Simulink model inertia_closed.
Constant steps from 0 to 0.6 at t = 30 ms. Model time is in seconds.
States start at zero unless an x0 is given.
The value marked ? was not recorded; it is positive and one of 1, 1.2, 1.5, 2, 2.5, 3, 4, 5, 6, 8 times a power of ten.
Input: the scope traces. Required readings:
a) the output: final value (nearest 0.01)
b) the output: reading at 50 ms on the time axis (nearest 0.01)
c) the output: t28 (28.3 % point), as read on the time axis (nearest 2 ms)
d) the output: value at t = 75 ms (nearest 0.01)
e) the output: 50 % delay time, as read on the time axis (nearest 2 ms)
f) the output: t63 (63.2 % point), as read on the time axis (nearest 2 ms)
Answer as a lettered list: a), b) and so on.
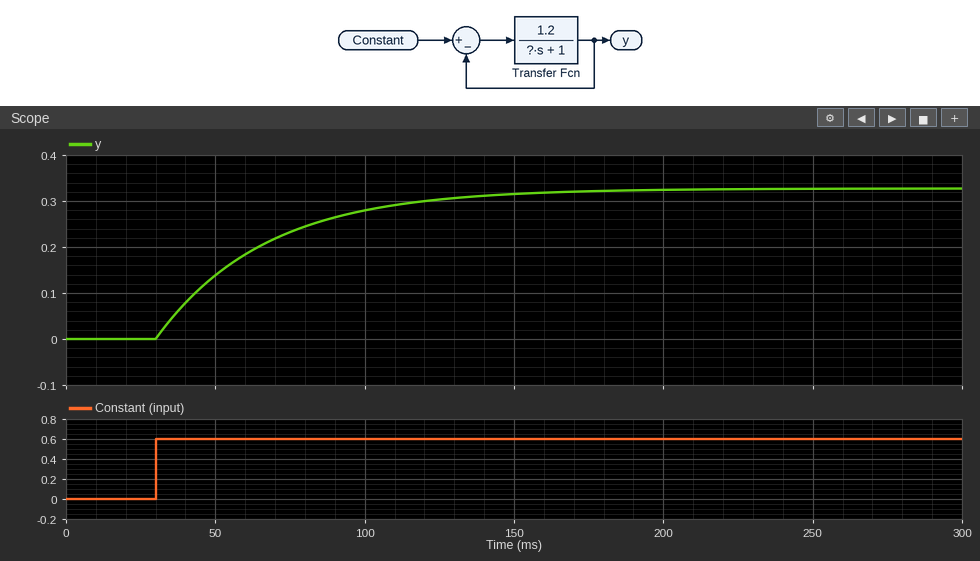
a) 0.33
b) 0.14
c) 42 ms
d) 0.23
e) 56 ms
f) 66 ms
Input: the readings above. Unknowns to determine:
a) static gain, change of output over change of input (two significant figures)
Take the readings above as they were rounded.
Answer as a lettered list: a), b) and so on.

a) 0.55
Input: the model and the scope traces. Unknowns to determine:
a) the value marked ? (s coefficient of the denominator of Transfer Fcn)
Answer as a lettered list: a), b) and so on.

a) 0.08
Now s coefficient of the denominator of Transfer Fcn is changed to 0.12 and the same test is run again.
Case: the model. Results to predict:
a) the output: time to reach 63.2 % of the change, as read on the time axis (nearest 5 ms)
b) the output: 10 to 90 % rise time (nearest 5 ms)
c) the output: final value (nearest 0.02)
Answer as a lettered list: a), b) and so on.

a) 85 ms
b) 120 ms
c) 0.32
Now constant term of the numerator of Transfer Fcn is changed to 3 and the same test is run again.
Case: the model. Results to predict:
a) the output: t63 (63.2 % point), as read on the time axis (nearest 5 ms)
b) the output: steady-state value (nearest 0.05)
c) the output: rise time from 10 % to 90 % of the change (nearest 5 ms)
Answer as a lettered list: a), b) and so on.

a) 50 ms
b) 0.45
c) 45 ms
